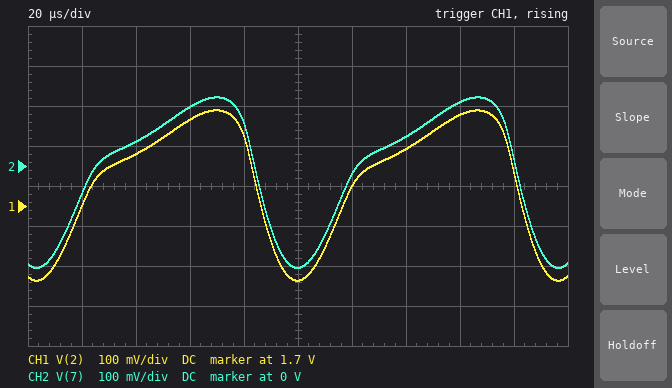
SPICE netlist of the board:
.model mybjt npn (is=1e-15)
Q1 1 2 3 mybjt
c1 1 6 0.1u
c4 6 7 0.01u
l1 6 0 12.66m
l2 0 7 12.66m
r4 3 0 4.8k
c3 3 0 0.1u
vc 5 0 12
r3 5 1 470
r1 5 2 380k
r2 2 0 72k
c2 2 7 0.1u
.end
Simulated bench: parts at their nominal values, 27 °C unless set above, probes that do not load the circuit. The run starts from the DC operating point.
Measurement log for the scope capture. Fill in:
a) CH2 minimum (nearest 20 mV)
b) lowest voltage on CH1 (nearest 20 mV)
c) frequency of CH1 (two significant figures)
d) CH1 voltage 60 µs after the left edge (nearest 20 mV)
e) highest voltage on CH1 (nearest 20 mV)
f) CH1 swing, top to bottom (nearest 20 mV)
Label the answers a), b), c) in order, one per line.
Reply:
a) -260 mV
b) 1.52 V
c) 10 kHz
d) 1.92 V
e) 1.94 V
f) 420 mV
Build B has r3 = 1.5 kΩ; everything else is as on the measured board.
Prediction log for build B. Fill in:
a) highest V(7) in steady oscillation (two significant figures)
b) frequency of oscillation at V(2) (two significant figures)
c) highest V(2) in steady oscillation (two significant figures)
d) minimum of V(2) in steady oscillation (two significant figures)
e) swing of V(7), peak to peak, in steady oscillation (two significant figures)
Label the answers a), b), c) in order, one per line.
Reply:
a) 490 mV
b) 9.5 kHz
c) 2.2 V
d) 1.0 V
e) 1.2 V
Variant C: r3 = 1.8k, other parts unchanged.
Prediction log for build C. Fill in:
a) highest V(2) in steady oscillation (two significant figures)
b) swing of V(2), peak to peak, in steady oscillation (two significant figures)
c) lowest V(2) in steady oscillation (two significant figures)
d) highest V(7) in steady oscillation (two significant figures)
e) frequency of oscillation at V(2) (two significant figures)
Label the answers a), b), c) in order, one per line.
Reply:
a) 2.4 V
b) 1.6 V
c) 800 mV
d) 630 mV
e) 9.5 kHz
